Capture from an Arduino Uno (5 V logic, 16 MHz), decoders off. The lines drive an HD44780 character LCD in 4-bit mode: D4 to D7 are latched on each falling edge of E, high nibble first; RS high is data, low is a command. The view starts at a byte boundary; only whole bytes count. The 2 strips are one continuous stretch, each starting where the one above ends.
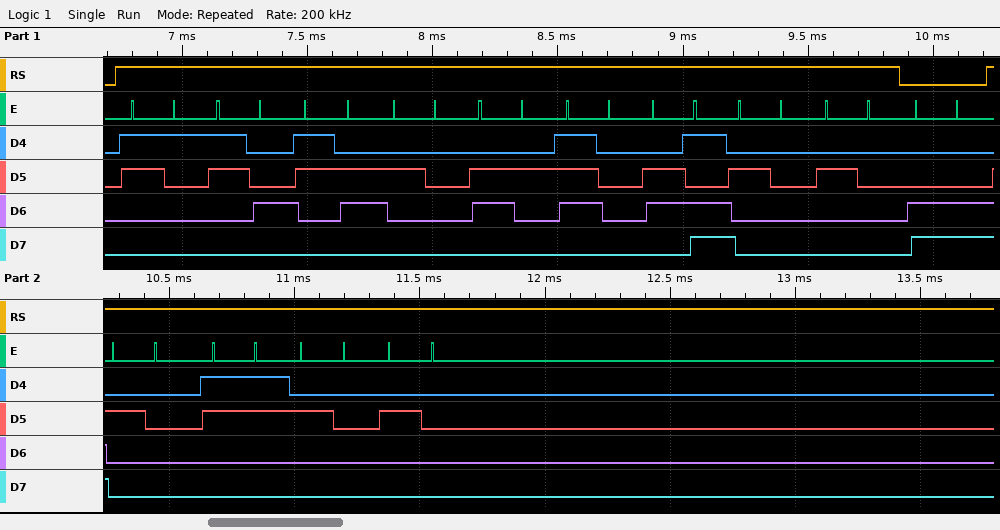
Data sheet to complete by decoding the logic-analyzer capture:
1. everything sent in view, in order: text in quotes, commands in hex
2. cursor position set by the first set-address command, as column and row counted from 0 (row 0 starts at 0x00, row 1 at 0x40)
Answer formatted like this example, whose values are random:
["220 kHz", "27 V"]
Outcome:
["\"146 bpm  \" 0xCC \" 3  \"", "column 12, row 1"]
